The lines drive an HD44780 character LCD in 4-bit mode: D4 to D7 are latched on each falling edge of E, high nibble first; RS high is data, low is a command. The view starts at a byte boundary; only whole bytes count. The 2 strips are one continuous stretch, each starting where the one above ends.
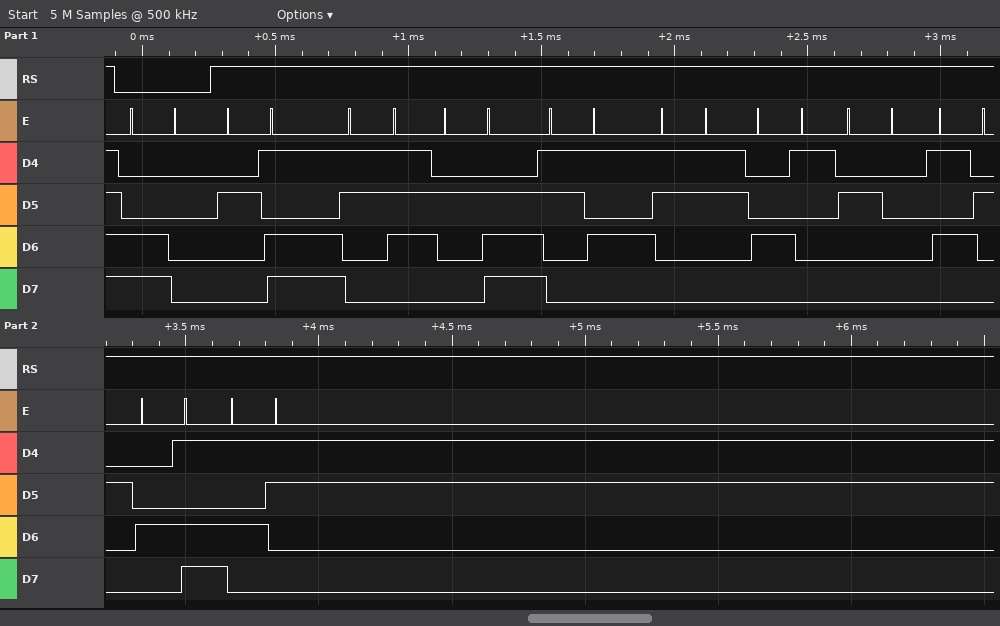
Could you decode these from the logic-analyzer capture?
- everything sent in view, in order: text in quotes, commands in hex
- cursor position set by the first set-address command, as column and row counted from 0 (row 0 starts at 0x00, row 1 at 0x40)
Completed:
0xC0 "-7.53A RMS"
column 0, row 1
